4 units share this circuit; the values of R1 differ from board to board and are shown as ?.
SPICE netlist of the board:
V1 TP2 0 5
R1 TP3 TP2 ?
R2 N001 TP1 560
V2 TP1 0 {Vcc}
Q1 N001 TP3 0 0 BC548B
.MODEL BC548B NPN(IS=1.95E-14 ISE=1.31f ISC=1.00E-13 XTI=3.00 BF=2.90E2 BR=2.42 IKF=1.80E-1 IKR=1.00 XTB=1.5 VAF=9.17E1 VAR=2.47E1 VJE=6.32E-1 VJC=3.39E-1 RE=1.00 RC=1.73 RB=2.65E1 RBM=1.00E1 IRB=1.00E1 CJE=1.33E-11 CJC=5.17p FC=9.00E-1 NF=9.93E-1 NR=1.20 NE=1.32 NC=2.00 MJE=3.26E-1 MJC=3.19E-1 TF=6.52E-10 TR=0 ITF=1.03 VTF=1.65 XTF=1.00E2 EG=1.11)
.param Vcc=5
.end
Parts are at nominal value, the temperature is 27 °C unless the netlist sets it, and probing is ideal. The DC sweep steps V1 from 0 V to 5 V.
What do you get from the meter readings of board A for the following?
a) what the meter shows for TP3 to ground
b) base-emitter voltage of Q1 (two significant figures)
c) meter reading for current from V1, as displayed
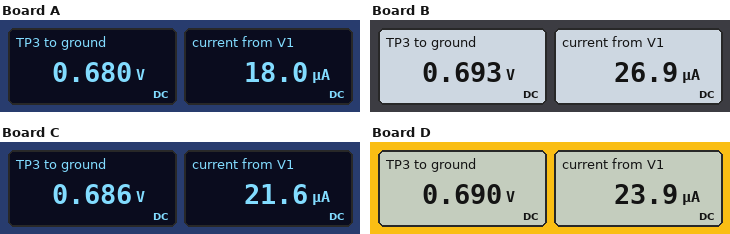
0.680 V
680 mV
18.0 µA
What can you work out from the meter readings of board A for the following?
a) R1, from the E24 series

240 kΩ
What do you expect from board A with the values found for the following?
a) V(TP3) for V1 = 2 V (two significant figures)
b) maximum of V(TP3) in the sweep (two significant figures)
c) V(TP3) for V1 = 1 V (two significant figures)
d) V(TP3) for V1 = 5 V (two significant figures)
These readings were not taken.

650 mV
680 mV
610 mV
680 mV
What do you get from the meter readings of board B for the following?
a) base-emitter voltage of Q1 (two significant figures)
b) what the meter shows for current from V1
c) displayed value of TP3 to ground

690 mV
26.9 µA
0.693 V
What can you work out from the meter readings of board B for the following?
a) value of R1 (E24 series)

160 kΩ
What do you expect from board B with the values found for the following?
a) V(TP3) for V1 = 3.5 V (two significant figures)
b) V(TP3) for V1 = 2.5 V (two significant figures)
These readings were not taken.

680 mV
670 mV
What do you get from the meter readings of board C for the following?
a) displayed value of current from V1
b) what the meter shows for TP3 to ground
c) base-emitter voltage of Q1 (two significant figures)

21.6 µA
0.686 V
690 mV
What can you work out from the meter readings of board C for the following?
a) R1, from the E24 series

200 kΩ
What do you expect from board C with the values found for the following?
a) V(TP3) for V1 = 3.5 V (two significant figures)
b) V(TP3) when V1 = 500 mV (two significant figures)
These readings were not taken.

670 mV
500 mV
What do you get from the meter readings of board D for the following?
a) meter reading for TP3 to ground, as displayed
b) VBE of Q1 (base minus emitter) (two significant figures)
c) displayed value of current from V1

0.690 V
690 mV
23.9 µA
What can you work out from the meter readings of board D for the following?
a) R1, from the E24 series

180 kΩ
